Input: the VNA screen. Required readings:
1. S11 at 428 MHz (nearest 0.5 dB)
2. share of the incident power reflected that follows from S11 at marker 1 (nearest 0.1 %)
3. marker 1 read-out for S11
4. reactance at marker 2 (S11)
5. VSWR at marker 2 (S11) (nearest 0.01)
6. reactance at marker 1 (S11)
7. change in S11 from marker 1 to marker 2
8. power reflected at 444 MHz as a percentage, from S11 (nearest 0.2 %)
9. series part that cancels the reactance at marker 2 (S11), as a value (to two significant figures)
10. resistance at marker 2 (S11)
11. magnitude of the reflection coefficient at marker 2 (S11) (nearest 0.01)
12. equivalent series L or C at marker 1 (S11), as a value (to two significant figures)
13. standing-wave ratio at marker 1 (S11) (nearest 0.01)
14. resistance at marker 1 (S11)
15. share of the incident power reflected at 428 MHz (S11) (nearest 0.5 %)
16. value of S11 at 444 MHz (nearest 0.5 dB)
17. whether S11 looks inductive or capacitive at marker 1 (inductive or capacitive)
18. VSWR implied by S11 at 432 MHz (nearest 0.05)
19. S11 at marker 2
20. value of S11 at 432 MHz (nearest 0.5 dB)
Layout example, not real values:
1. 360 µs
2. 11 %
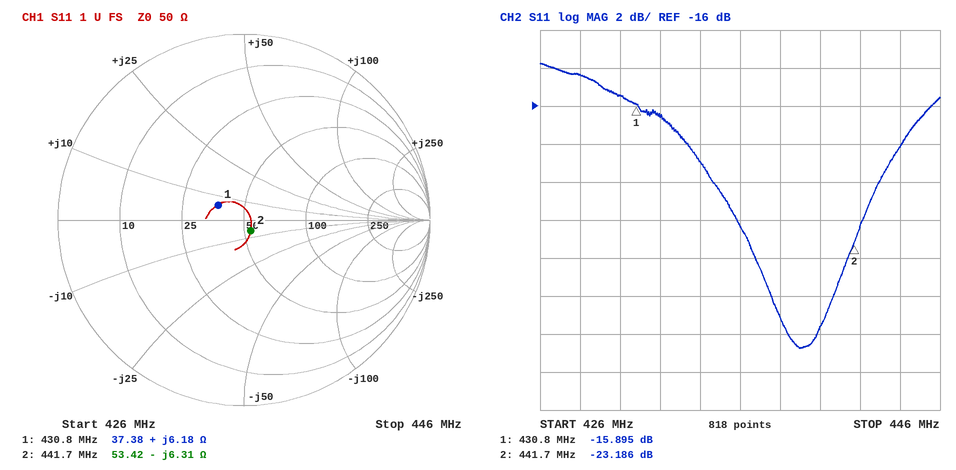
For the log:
1. -14.5 dB
2. 2.6 %
3. -15.895 dB
4. -6.31 Ω
5. 1.15
6. +6.18 Ω
7. -7.291 dB
8. 1.6 %
9. 2.3 nH
10. 53.42 Ω
11. 0.07
12. 2.3 nH
13. 1.38
14. 37.38 Ω
15. 3.5 %
16. -18.0 dB
17. inductive
18. 1.35
19. -23.186 dB
20. -16.5 dB
